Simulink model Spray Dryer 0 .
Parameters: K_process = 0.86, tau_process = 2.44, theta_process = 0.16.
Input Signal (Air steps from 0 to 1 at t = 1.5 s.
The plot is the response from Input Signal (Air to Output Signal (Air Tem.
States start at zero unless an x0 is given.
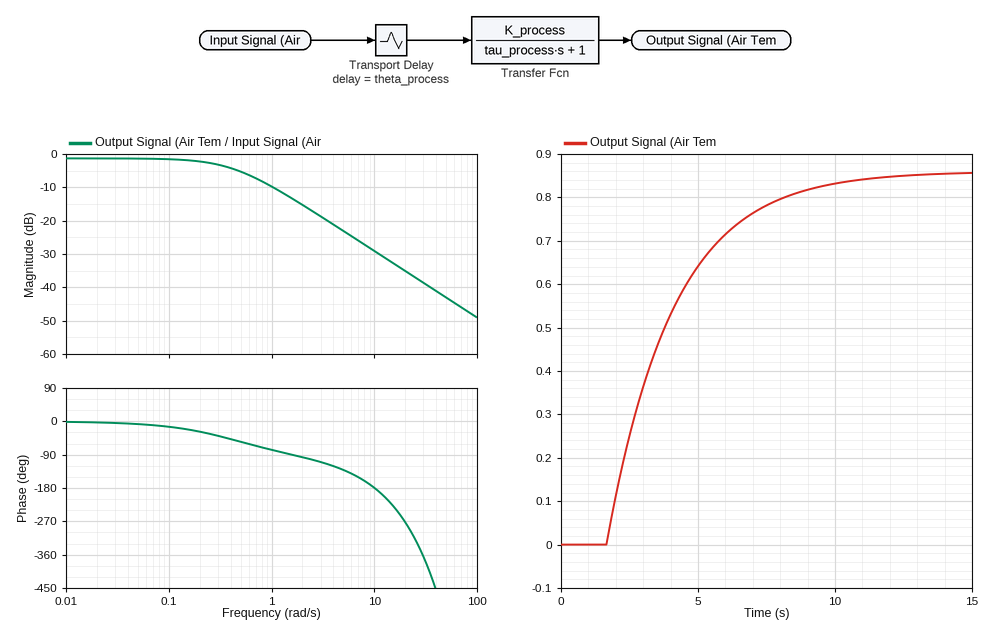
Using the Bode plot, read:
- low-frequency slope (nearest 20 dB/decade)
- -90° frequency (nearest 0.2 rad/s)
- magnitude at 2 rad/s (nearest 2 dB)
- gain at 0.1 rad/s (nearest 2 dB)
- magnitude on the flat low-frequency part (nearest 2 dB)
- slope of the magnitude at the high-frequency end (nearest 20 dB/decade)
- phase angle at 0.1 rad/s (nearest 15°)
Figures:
0 dB/decade
1.6 rad/s
-16 dB
-2 dB
-2 dB
-20 dB/decade
-15°
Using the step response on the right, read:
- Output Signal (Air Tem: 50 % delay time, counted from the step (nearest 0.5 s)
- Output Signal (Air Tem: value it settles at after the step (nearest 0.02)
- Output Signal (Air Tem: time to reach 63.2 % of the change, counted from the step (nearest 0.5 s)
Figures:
2.0 s
0.86
2.5 s
